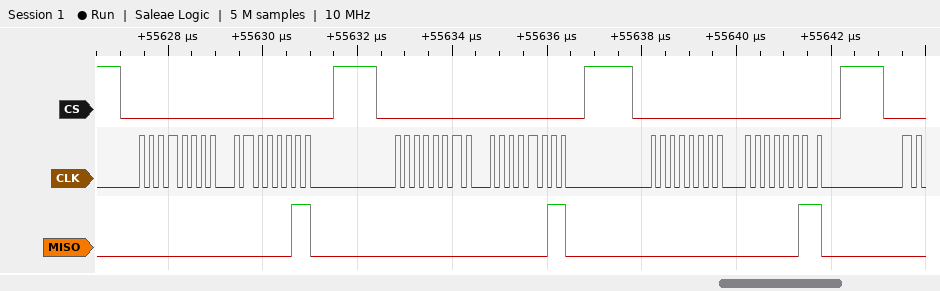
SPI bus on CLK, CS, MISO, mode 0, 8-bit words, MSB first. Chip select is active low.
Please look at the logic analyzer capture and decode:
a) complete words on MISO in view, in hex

00, 03, 00, 03, 00, 03
